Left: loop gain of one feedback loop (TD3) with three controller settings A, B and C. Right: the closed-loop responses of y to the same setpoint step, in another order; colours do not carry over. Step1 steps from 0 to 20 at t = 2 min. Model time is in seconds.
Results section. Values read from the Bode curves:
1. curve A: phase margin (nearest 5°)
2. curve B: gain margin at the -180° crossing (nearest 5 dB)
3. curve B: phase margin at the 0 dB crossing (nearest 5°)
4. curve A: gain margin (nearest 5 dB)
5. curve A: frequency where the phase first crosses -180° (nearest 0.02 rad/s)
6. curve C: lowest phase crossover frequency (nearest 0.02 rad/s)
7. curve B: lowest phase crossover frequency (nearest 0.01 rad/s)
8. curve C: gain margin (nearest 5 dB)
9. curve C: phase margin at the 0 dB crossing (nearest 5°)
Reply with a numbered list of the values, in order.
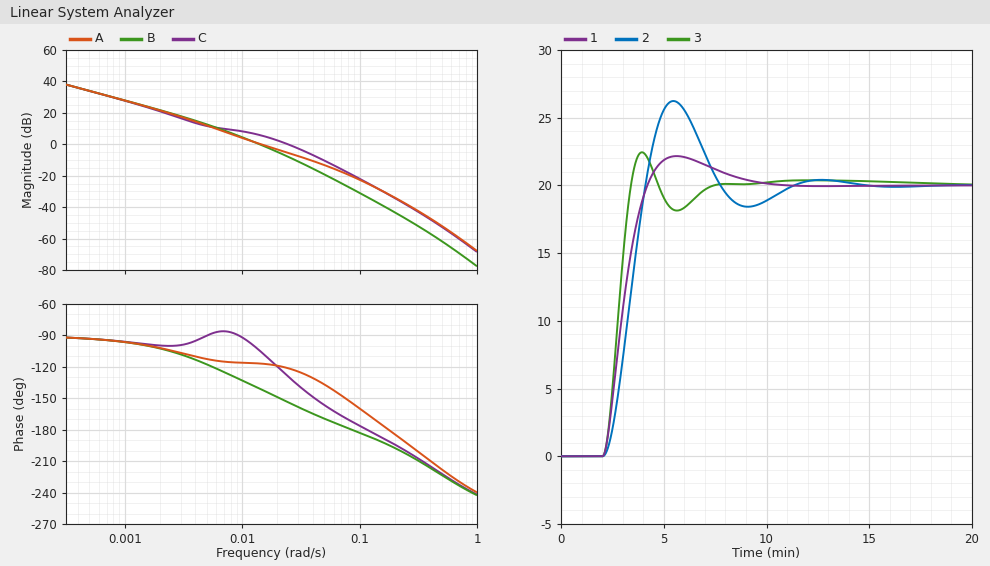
1. 65°
2. 30 dB
3. 40°
4. 30 dB
5. 0.18 rad/s
6. 0.12 rad/s
7. 0.09 rad/s
8. 25 dB
9. 50°
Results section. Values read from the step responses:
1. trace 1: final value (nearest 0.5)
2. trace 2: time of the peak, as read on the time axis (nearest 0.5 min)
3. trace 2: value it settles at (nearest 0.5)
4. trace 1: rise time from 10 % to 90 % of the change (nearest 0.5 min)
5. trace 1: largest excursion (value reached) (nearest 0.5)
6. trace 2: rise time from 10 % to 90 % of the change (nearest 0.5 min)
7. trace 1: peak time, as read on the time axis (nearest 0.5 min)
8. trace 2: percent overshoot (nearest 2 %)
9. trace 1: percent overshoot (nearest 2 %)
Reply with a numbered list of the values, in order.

1. 20.0
2. 5.5 min
3. 20.0
4. 1.5 min
5. 22.0
6. 1.5 min
7. 5.5 min
8. 32 %
9. 10 %
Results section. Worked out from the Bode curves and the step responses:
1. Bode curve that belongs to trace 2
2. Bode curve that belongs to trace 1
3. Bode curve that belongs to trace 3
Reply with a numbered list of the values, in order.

1. B
2. A
3. C
